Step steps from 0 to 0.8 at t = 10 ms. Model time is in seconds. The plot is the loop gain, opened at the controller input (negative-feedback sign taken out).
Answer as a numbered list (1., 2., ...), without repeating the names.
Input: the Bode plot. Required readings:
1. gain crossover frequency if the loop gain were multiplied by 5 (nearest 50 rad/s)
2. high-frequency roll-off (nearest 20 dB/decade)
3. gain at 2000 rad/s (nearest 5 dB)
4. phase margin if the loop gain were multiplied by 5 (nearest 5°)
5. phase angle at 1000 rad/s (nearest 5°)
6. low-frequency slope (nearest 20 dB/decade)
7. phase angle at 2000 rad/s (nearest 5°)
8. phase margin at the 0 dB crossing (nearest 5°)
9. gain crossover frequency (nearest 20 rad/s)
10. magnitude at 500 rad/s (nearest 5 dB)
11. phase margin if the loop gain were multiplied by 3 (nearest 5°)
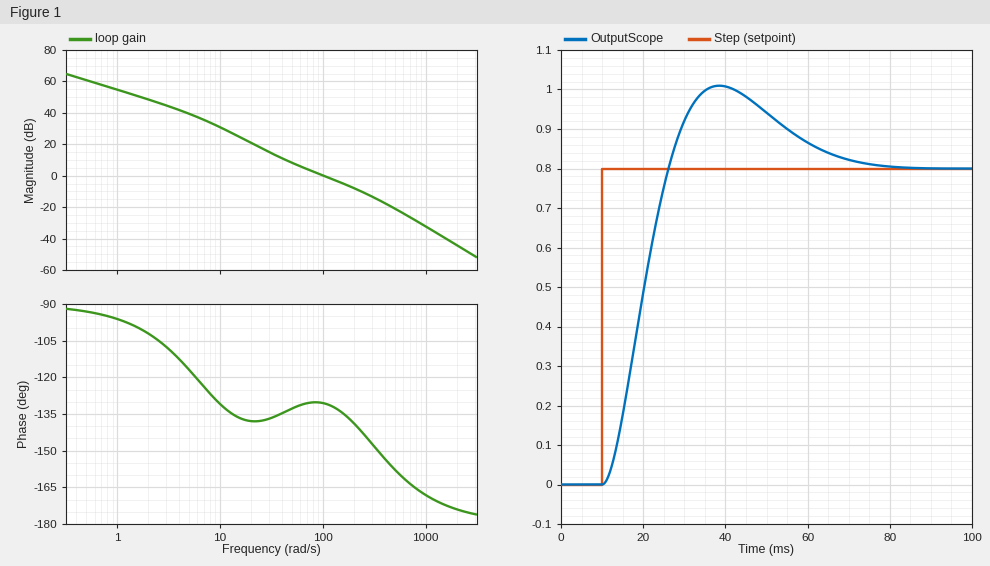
1. 300 rad/s
2. -40 dB/decade
3. -45 dB
4. 30°
5. -170°
6. -20 dB/decade
7. -175°
8. 50°
9. 100 rad/s
10. -20 dB
11. 40°
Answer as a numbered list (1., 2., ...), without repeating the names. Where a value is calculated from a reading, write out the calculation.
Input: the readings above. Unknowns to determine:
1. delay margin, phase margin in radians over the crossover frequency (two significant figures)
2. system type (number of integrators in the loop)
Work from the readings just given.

1. 50 × π / 180 / 100 = 0.0087 s
2. 1
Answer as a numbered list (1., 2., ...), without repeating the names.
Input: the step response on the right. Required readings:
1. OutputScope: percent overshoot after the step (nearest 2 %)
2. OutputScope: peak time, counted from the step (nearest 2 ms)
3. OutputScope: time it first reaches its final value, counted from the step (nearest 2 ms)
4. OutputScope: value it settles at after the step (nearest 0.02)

1. 26 %
2. 28 ms
3. 16 ms
4. 0.80
